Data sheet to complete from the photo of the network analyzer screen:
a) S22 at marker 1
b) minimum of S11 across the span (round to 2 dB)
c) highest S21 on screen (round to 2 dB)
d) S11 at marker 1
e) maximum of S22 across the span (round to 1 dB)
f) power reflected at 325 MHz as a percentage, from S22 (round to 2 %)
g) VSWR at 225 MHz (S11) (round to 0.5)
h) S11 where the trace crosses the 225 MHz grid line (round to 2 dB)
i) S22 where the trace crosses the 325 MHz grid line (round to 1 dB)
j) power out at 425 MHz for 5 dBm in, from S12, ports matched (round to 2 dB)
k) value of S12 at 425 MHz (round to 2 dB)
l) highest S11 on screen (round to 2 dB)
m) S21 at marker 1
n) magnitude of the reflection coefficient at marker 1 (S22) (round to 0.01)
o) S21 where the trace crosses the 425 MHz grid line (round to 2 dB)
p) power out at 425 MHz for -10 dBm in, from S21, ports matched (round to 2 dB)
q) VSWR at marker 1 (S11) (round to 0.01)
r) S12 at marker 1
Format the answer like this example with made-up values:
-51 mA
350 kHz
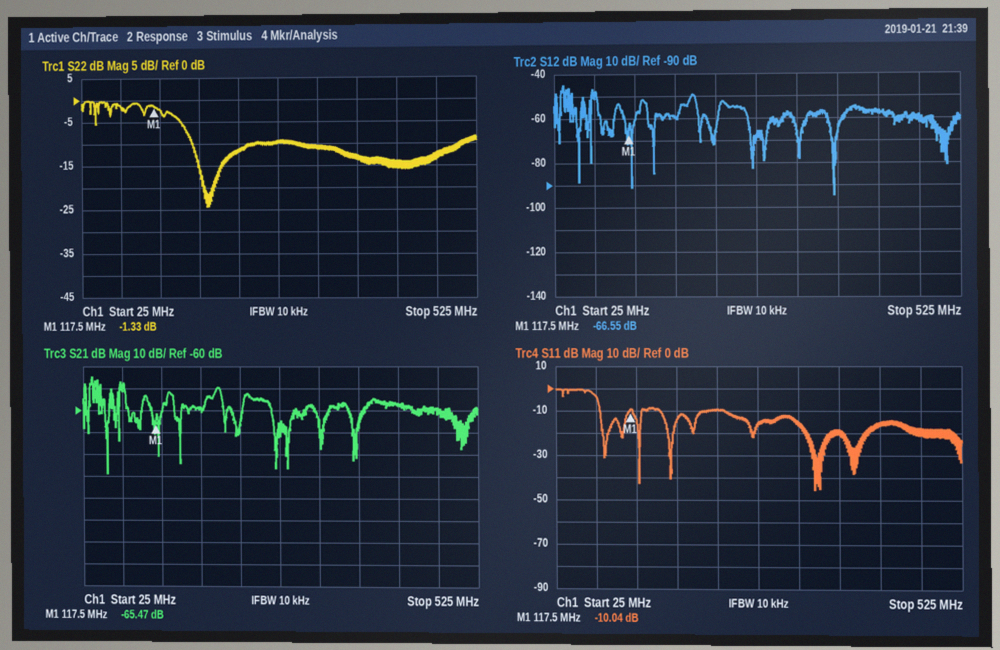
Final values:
-1.33 dB
-46 dB
-44 dB
-10.04 dB
0 dB
8 %
2.0
-10 dB
-11 dB
-52 dBm
-58 dB
0 dB
-65.47 dB
0.86
-58 dB
-68 dBm
1.92
-66.55 dB
